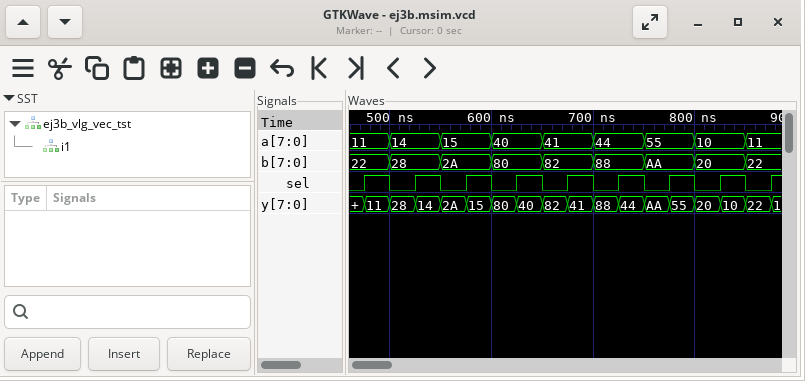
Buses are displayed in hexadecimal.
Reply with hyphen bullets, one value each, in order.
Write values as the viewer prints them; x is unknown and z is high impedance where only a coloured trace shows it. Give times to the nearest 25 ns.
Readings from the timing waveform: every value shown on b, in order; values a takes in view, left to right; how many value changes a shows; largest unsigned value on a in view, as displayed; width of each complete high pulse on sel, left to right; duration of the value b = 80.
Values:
- 22, 28, 2A, 80, 82, 88, AA, 20, 22
- 11, 14, 15, 40, 41, 44, 55, 10, 11
- 8
- 55
- 25 ns, 25 ns, 25 ns, 25 ns, 25 ns, 25 ns, 25 ns, 25 ns
- 50 ns
